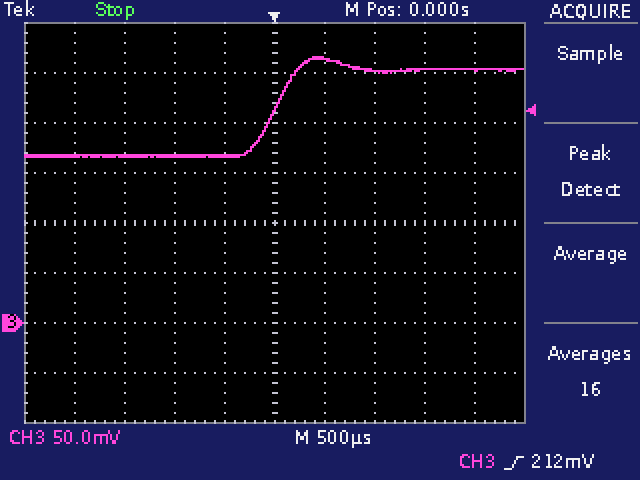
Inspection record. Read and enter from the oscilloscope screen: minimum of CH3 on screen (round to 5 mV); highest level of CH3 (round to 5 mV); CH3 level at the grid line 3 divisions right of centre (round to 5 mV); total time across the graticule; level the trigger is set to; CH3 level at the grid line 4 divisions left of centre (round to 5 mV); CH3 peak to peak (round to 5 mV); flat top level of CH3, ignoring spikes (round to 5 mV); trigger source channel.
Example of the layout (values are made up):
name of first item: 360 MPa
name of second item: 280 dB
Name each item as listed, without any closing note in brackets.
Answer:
minimum of CH3 on screen: 165 mV
highest level of CH3: 265 mV
CH3 level at the grid line 3 divisions right of centre: 255 mV
total time across the graticule: 5 ms
level the trigger is set to: 212 mV
CH3 level at the grid line 4 divisions left of centre: 165 mV
CH3 peak to peak: 100 mV
flat top level of CH3, ignoring spikes: 255 mV
trigger source channel: CH3
